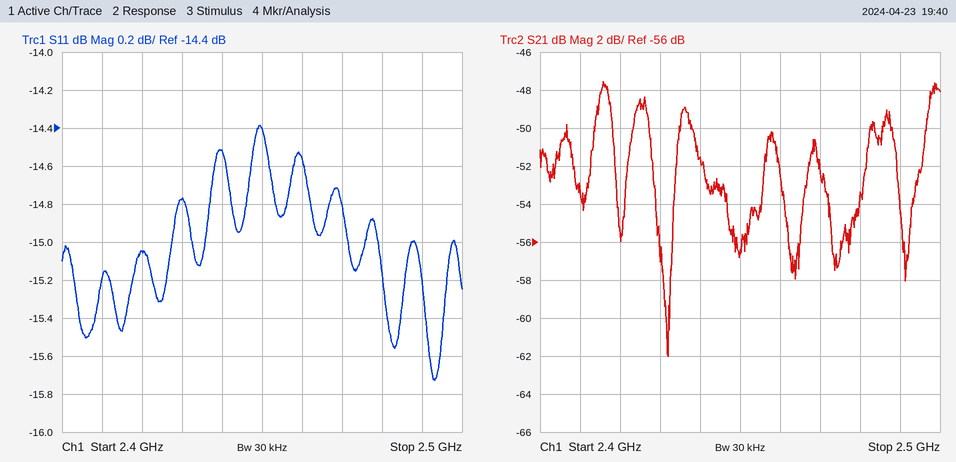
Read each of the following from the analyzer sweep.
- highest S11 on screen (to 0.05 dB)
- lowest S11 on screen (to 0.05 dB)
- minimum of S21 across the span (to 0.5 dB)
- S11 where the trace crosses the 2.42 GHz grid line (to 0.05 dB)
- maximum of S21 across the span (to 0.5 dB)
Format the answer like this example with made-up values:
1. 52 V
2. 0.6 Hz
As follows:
1. -14.40 dB
2. -15.75 dB
3. -62.0 dB
4. -15.05 dB
5. -47.5 dB
